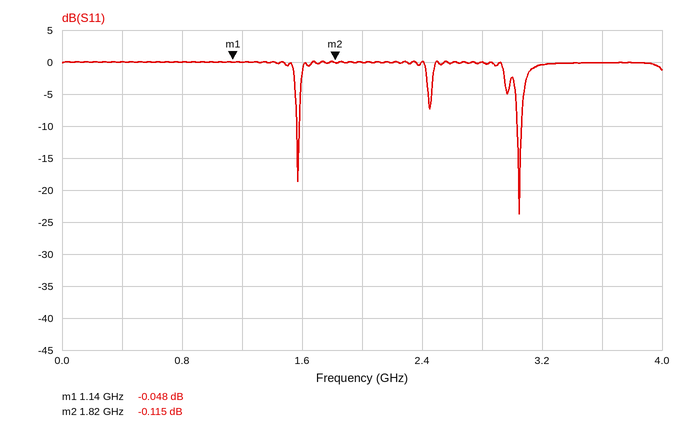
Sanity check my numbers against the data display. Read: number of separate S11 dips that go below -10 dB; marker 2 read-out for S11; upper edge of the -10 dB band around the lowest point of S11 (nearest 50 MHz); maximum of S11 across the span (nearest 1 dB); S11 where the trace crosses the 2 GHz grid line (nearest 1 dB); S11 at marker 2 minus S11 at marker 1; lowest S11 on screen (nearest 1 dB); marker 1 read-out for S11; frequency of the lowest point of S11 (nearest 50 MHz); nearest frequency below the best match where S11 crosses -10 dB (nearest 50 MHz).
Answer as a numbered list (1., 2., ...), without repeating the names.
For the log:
1. 2
2. -0.115 dB
3. 3.05 GHz
4. 0 dB
5. 0 dB
6. -0.067 dB
7. -24 dB
8. -0.048 dB
9. 3.05 GHz
10. 3.05 GHz
